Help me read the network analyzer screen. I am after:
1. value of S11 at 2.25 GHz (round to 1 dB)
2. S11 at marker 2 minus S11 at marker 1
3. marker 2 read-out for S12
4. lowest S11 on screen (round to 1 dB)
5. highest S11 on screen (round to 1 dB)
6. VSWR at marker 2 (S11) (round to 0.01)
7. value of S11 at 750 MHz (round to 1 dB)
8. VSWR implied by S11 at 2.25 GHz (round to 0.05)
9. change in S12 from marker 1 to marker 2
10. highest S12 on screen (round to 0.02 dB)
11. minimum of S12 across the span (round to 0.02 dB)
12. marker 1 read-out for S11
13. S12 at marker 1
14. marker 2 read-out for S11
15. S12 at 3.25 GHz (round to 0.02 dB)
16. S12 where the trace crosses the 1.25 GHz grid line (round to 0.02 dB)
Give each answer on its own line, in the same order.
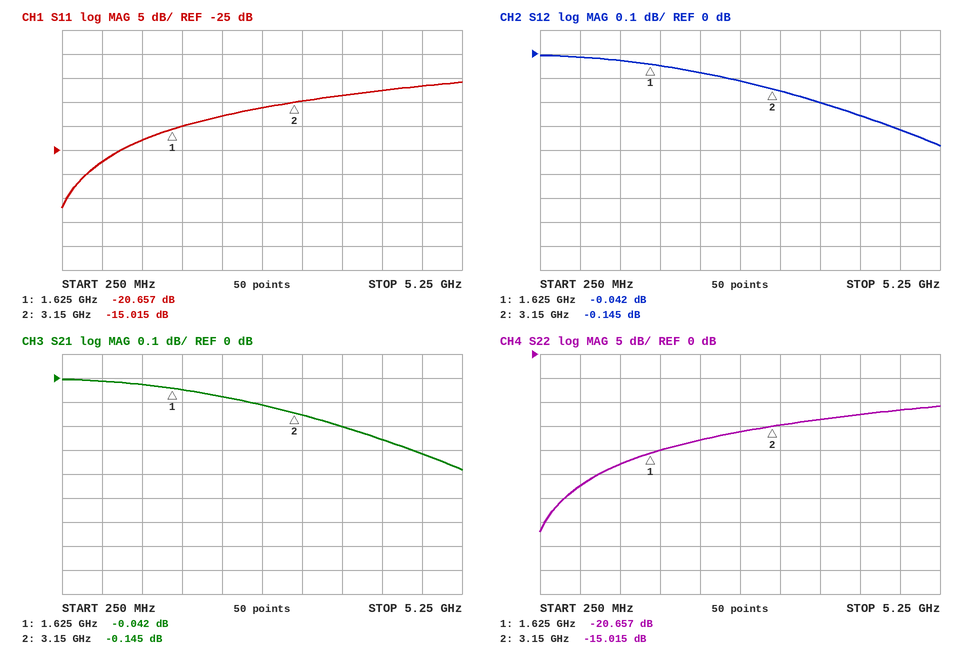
-18 dB
5.642 dB
-0.145 dB
-37 dB
-11 dB
1.43
-27 dB
1.30
-0.103 dB
0.00 dB
-0.38 dB
-20.657 dB
-0.042 dB
-15.015 dB
-0.16 dB
-0.02 dB
